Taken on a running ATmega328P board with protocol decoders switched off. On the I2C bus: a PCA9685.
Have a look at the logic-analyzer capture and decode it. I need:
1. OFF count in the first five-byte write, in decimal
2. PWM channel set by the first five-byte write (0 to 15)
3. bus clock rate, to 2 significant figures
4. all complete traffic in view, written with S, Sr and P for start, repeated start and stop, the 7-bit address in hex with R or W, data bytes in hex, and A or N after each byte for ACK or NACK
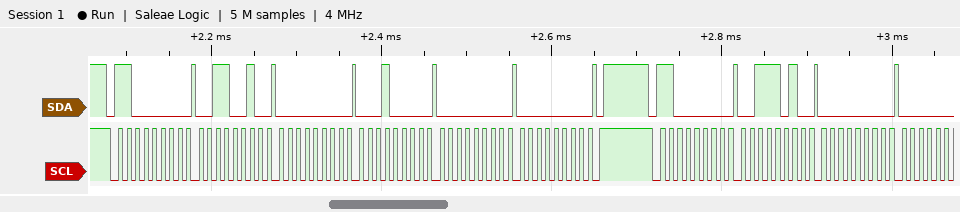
0
11
100 kHz
S 60W A 32 A 00 A 10 A 00 A 00 A P S 60W A 3A A 00 A
